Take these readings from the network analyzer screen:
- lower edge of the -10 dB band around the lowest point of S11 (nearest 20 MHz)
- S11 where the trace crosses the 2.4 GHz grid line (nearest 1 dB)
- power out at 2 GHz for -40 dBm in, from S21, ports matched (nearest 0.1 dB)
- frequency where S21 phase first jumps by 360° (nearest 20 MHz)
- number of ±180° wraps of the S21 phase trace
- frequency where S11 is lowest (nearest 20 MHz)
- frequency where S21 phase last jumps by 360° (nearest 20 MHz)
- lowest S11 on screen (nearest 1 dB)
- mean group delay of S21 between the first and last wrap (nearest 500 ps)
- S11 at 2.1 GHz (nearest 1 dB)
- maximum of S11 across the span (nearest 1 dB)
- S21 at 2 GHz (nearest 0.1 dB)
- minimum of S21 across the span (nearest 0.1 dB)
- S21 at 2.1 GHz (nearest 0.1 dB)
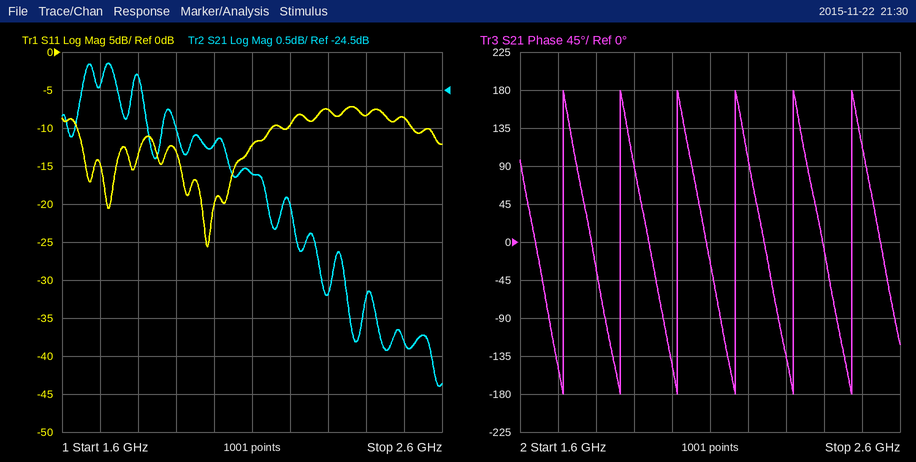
1.64 GHz
-8 dB
-65.2 dBm
1.72 GHz
6
1.98 GHz
2.48 GHz
-26 dB
6.5 ns
-12 dB
-7 dB
-25.2 dB
-28.4 dB
-25.6 dB
